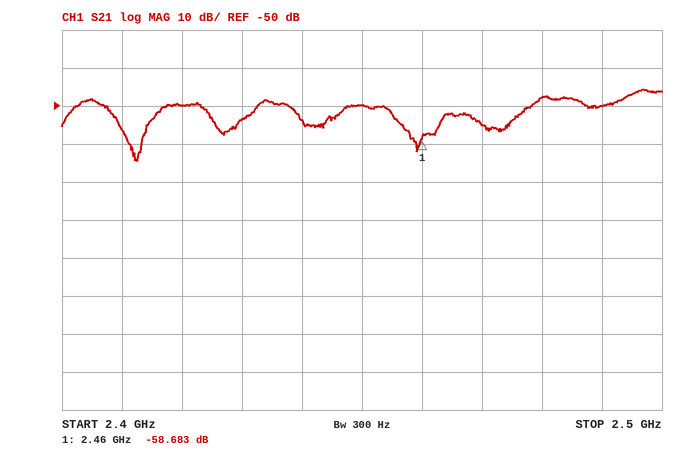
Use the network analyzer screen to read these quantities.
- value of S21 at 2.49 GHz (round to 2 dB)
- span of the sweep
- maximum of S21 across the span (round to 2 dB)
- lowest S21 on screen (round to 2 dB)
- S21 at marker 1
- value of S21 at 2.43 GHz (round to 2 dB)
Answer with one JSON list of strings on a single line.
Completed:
["-50 dB", "100 MHz", "-46 dB", "-64 dB", "-58.683 dB", "-54 dB"]
